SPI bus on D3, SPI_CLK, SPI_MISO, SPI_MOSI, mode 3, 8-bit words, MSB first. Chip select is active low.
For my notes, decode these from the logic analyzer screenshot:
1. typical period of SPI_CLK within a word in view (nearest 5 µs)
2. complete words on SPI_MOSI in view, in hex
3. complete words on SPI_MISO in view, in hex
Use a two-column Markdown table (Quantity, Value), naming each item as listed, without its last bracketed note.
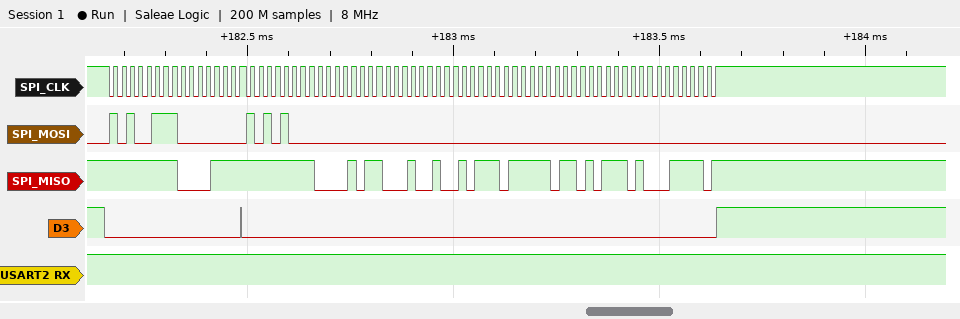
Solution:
| Quantity | Value |
|---|---|
| typical period of SPI_CLK within a word in view | 20 µs |
| complete words on SPI_MOSI in view, in hex | A7, 00, A8, 00, 00, 00, 00, 00, 00 |
| complete words on SPI_MISO in view, in hex | FF, 0F, FF, 0B, 12, 5D, F6, BA, 3D |
